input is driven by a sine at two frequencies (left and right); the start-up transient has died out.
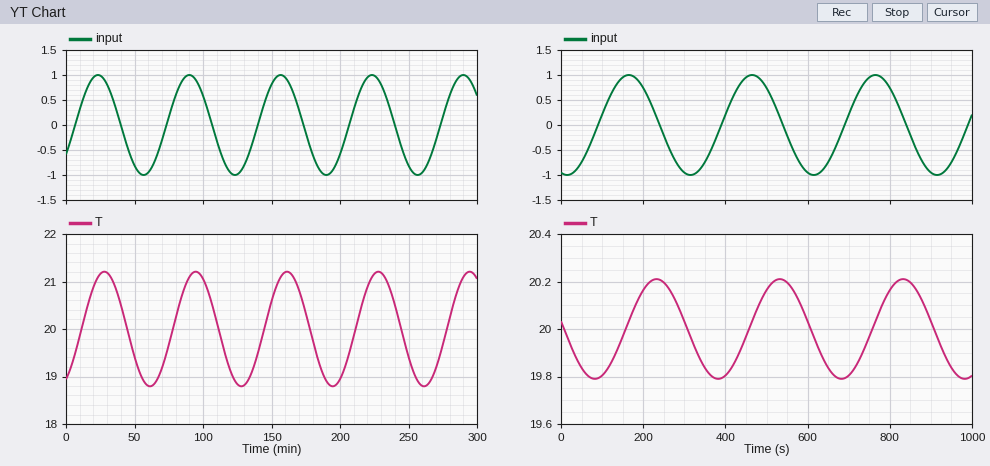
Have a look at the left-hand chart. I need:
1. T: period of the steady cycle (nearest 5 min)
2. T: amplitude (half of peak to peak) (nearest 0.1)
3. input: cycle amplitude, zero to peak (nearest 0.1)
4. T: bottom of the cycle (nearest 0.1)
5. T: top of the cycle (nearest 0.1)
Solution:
65 min
1.2
1.0
18.8
21.2
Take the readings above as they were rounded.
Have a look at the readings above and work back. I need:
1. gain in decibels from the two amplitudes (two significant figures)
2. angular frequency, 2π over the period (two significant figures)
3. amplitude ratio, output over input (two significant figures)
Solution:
1.6 dB
0.097 rad/min
1.2
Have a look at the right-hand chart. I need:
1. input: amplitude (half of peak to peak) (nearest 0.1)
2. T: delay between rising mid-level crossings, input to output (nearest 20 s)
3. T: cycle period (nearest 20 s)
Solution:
1.0
60 s
300 s
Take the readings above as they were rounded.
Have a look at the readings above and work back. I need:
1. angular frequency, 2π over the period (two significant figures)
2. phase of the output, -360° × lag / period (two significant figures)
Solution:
0.021 rad/s
-72°
